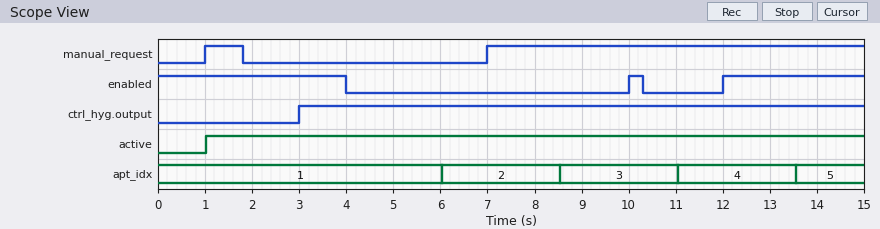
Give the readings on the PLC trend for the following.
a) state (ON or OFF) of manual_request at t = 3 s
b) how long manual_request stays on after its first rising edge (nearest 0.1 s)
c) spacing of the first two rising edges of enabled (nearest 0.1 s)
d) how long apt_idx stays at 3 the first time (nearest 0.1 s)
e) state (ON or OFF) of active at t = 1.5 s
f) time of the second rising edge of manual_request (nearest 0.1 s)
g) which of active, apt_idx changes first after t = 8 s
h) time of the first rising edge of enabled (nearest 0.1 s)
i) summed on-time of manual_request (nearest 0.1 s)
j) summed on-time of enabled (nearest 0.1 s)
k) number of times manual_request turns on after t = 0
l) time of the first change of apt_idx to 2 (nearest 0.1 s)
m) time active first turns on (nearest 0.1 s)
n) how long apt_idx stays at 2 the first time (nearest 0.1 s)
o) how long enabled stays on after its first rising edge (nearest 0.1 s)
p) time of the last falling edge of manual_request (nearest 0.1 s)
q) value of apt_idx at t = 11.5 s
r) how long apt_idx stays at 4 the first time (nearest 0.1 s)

OFF
0.8 s
2.0 s
2.5 s
ON
7.0 s
apt_idx
10.0 s
8.8 s
7.3 s
2
6.0 s
1.0 s
2.5 s
0.3 s
1.8 s
4
2.5 s
